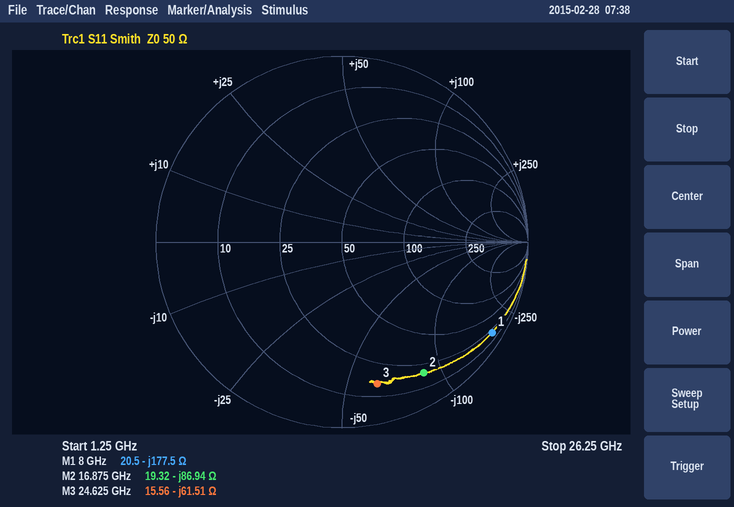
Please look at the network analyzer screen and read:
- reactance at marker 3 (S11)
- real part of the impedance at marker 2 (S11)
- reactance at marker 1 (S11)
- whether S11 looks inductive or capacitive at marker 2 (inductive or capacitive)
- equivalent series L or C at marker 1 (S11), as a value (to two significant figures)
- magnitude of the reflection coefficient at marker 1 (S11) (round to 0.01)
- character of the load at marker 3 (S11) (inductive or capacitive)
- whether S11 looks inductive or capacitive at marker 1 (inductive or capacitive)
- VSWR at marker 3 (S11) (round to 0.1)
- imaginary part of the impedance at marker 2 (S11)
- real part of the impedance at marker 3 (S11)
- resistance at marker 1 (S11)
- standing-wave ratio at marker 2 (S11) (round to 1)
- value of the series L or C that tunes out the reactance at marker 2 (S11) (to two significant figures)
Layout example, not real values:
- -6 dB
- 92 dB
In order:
- -61.51 Ω
- 19.32 Ω
- -177.5 Ω
- capacitive
- 110 fF
- 0.94
- capacitive
- capacitive
- 8.3
- -86.94 Ω
- 15.56 Ω
- 20.5 Ω
- 11
- 820 pH
